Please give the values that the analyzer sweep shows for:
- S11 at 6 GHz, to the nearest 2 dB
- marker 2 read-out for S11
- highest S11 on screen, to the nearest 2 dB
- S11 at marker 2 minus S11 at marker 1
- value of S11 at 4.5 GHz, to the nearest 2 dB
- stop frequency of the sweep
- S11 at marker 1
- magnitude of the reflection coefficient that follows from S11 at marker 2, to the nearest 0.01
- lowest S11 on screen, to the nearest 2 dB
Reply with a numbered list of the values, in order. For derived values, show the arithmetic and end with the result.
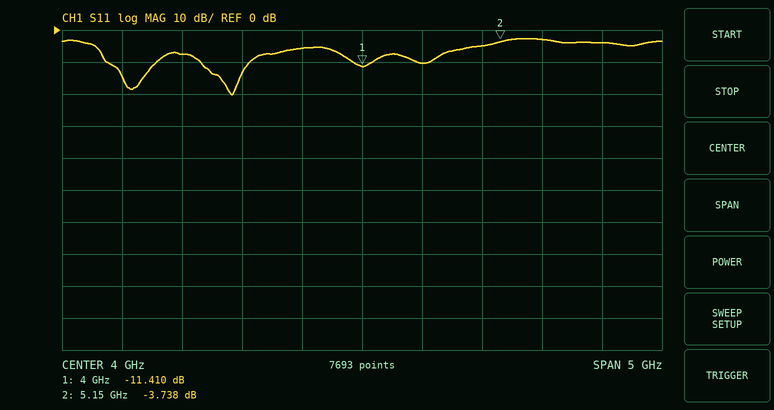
1. -4 dB
2. -3.738 dB
3. -2 dB
4. -3.738 − (-11.41) = 7.672 dB
5. -10 dB
6. 6.5 GHz
7. -11.410 dB
8. 10^(-3.738/20) ≈ 0.65
9. -20 dB
